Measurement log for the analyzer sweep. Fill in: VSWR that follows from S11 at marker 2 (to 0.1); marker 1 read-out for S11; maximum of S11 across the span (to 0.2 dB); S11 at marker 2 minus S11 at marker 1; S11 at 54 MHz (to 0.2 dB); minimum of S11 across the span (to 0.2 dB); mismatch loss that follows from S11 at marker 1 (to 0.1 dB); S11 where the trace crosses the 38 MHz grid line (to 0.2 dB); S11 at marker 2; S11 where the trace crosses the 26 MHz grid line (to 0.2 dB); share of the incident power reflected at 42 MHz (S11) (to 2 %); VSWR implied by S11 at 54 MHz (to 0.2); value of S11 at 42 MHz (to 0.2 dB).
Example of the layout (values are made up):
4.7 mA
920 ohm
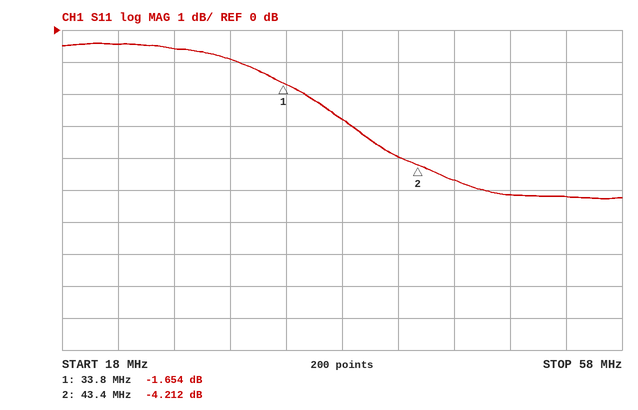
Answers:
4.2
-1.654 dB
-0.4 dB
-2.558 dB
-5.2 dB
-5.2 dB
5.0 dB
-2.8 dB
-4.212 dB
-0.6 dB
40 %
3.4
-4.0 dB
